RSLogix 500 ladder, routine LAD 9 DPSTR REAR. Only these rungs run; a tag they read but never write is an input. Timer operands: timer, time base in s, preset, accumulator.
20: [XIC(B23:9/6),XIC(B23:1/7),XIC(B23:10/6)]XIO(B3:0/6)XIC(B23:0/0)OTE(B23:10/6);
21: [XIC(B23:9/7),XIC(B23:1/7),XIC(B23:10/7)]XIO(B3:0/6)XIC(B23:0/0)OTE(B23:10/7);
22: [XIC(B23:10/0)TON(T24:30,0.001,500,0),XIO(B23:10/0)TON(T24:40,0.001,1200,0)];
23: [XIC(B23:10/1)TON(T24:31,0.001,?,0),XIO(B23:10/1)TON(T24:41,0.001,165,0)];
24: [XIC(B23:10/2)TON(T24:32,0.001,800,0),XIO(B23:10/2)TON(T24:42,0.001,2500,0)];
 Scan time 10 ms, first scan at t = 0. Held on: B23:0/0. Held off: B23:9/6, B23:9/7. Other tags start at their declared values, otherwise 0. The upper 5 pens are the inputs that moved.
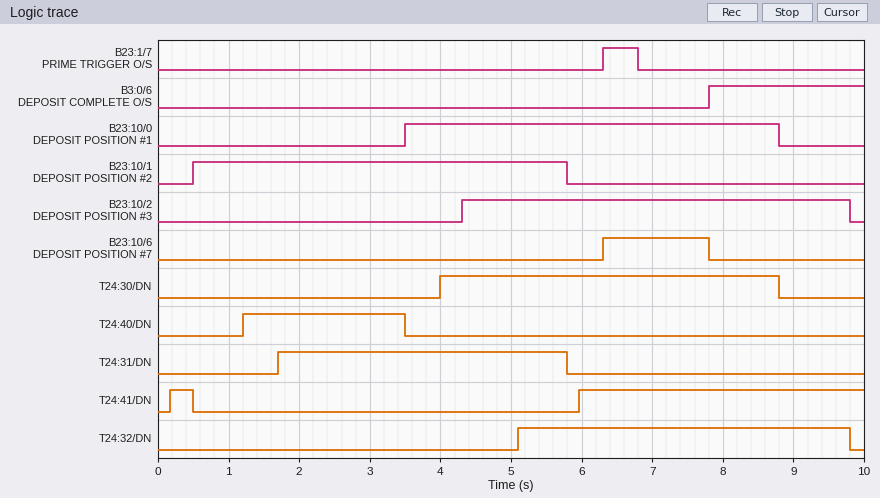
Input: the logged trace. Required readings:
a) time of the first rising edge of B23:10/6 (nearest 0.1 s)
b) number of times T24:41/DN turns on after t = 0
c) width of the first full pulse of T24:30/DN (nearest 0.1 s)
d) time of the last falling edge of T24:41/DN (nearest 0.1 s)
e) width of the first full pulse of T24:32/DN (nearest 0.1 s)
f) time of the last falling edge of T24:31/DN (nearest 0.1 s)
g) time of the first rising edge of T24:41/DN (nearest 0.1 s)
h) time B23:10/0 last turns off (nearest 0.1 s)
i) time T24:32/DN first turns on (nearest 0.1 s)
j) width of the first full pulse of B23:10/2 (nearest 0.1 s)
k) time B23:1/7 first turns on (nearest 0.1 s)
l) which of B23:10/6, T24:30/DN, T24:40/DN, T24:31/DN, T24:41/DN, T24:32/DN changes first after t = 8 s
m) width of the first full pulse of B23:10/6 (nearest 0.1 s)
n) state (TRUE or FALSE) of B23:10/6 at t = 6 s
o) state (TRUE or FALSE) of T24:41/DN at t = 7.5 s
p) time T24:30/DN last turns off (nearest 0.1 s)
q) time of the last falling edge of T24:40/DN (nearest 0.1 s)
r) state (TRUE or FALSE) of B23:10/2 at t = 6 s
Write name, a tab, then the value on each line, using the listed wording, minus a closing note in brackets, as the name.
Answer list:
time of the first rising edge of B23:10/6	6.3 s
number of times T24:41/DN turns on after t = 0	2
width of the first full pulse of T24:30/DN	4.8 s
time of the last falling edge of T24:41/DN	0.5 s
width of the first full pulse of T24:32/DN	4.7 s
time of the last falling edge of T24:31/DN	5.8 s
time of the first rising edge of T24:41/DN	0.2 s
time B23:10/0 last turns off	8.8 s
time T24:32/DN first turns on	5.1 s
width of the first full pulse of B23:10/2	5.5 s
time B23:1/7 first turns on	6.3 s
which of B23:10/6, T24:30/DN, T24:40/DN, T24:31/DN, T24:41/DN, T24:32/DN changes first after t = 8 s	T24:30/DN
width of the first full pulse of B23:10/6	1.5 s
state (TRUE or FALSE) of B23:10/6 at t = 6 s	FALSE
state (TRUE or FALSE) of T24:41/DN at t = 7.5 s	TRUE
time T24:30/DN last turns off	8.8 s
time of the last falling edge of T24:40/DN	3.5 s
state (TRUE or FALSE) of B23:10/2 at t = 6 s	TRUE
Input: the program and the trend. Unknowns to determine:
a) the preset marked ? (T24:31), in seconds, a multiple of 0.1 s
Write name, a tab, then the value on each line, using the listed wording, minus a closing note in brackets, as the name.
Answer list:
the preset marked ? (T24:31), in seconds, a multiple of 0.1 s	1.2 s
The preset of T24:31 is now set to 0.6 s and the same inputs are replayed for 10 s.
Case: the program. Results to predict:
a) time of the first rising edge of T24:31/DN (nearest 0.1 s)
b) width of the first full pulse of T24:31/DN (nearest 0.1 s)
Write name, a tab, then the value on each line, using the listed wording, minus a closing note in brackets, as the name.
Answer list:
time of the first rising edge of T24:31/DN	1.1 s
width of the first full pulse of T24:31/DN	4.7 s
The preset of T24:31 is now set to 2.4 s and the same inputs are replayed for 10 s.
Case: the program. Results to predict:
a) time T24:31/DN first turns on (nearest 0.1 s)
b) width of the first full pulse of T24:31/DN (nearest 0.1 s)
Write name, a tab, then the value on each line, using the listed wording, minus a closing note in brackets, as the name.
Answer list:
time T24:31/DN first turns on	2.9 s
width of the first full pulse of T24:31/DN	2.9 s
